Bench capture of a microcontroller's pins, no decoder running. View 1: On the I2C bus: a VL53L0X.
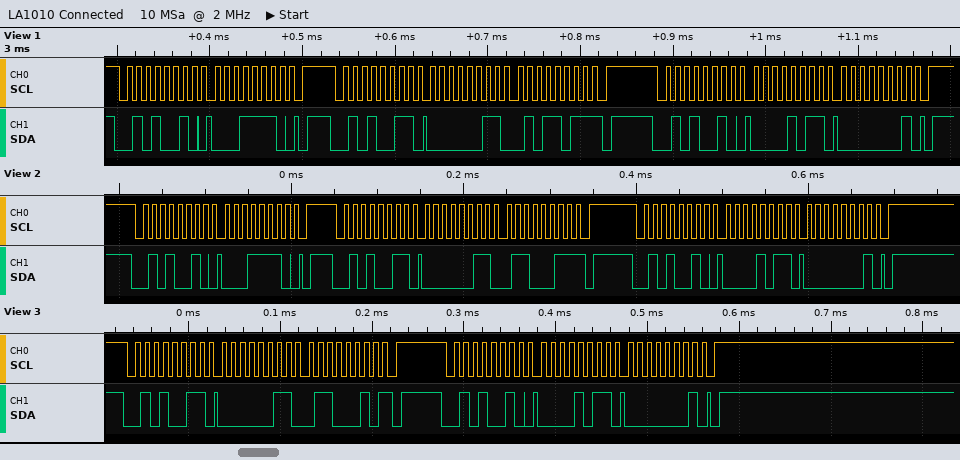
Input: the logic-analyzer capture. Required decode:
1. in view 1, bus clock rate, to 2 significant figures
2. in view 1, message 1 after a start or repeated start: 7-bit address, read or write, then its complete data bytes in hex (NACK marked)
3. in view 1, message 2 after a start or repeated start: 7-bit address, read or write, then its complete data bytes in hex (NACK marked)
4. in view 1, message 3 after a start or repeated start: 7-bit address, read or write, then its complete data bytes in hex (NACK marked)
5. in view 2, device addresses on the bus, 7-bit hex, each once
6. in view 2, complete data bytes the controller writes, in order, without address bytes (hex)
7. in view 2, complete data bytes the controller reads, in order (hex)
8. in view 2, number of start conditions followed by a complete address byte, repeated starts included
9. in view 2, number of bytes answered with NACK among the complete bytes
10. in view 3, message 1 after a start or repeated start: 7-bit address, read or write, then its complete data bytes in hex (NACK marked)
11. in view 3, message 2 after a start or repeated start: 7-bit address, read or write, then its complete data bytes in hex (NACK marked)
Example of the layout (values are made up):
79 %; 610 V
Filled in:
100 kHz; 0x29 write: 1E; 0x29 read: 03 5B NACK; 0x29 write: 0B 01; 0x29; 1E 0B 01; 03 63; 3; 1; 0x29 read: 03 62 NACK; 0x29 write: 0B 01
